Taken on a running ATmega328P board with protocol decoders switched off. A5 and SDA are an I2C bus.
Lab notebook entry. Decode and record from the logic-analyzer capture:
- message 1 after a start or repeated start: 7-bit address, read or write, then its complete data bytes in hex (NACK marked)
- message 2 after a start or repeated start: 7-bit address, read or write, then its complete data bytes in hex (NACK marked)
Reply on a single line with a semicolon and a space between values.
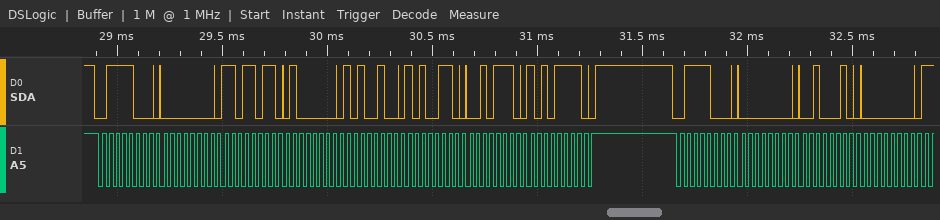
0x3C write: 00 DB 40 A4 A6 2E AF; 0x3C write: 00 22 00
